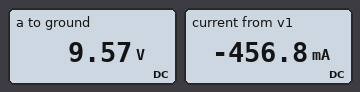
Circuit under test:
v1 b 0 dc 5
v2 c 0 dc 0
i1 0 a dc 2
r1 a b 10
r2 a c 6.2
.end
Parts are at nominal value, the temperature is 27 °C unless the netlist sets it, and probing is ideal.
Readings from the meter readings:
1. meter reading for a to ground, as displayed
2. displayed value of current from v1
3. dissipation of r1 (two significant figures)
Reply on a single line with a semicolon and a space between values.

9.57 V; -456.8 mA; 2.1 W
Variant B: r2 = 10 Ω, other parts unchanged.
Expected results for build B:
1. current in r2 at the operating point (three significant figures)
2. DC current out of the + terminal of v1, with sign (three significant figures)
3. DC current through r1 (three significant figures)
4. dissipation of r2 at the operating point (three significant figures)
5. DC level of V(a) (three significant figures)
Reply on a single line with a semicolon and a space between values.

1.25 A; -750 mA; 750 mA; 15.6 W; 12.5 V
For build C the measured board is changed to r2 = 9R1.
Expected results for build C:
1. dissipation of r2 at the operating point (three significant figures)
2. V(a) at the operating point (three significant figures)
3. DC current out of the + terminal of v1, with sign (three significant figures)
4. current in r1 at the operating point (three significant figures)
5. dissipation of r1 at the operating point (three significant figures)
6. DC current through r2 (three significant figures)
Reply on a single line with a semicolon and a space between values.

15.6 W; 11.9 V; -691 mA; 691 mA; 4.78 W; 1.31 A
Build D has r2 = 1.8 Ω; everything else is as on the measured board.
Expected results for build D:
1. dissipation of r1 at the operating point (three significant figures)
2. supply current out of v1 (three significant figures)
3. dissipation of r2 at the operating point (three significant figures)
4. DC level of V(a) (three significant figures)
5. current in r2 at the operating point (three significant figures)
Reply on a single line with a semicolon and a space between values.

141 mW; 119 mA; 8.08 W; 3.81 V; 2.12 A
